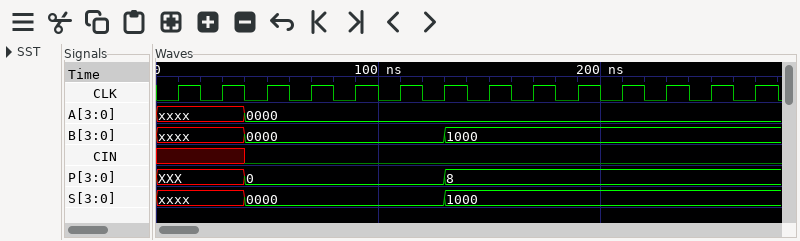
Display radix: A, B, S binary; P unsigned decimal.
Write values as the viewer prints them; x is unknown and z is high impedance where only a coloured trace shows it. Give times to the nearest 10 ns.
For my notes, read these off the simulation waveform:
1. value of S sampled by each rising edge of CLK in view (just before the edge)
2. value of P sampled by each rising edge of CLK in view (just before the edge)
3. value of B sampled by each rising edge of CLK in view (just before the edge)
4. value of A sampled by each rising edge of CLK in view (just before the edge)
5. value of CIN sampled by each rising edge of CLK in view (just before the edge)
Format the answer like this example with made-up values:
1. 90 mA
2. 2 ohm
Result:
1. xxxx, xxxx, 0000, 0000, 0000, 0000, 0000, 1000, 1000, 1000, 1000, 1000, 1000, 1000
2. XXX, XXX, 0, 0, 0, 0, 0, 8, 8, 8, 8, 8, 8, 8
3. xxxx, xxxx, 0000, 0000, 0000, 0000, 0000, 1000, 1000, 1000, 1000, 1000, 1000, 1000
4. xxxx, xxxx, 0000, 0000, 0000, 0000, 0000, 0000, 0000, 0000, 0000, 0000, 0000, 0000
5. x x 0 0 0 0 0 0 0 0 0 0 0 0
